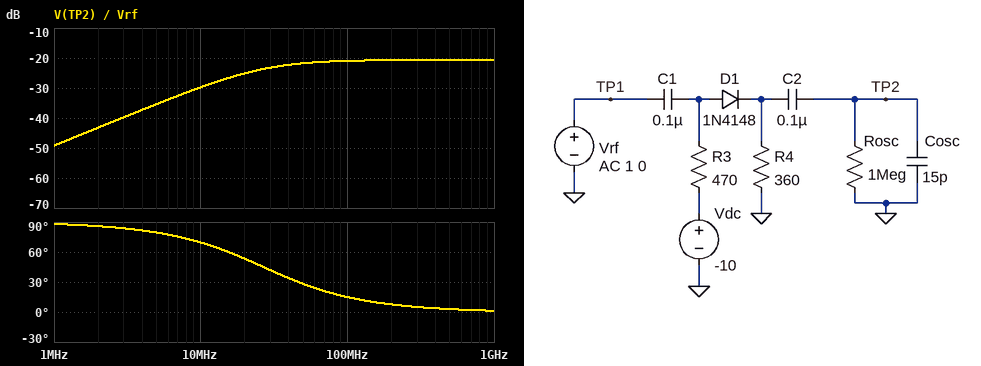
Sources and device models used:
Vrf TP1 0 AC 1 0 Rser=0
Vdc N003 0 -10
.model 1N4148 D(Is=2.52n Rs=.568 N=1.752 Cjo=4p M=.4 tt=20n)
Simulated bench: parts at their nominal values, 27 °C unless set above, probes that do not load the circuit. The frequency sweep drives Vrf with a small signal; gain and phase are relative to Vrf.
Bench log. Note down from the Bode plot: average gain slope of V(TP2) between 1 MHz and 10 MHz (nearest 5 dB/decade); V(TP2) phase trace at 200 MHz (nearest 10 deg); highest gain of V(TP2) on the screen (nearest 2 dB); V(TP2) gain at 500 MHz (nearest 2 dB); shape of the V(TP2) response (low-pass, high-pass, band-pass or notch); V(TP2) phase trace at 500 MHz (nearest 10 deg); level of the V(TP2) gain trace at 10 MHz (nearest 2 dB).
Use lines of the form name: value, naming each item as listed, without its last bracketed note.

average gain slope of V(TP2) between 1 MHz and 10 MHz: 20 dB/decade
V(TP2) phase trace at 200 MHz: 10 deg
highest gain of V(TP2) on the screen: -20 dB
V(TP2) gain at 500 MHz: -20 dB
shape of the V(TP2) response: high-pass
V(TP2) phase trace at 500 MHz: 0 deg
level of the V(TP2) gain trace at 10 MHz: -30 dB
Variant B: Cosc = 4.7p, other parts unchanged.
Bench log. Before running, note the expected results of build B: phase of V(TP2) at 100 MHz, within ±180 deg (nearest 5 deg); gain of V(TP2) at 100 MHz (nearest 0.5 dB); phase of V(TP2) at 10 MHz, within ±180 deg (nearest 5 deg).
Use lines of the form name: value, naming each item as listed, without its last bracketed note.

phase of V(TP2) at 100 MHz, within ±180 deg: 35 deg
gain of V(TP2) at 100 MHz: -14.0 dB
phase of V(TP2) at 10 MHz, within ±180 deg: 80 deg
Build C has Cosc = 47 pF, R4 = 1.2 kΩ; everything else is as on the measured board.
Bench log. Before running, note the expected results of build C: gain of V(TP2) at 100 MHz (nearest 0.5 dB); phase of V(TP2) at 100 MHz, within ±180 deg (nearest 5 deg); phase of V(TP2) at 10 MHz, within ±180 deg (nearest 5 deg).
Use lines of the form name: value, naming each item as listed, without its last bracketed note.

gain of V(TP2) at 100 MHz: -30.0 dB
phase of V(TP2) at 100 MHz, within ±180 deg: 0 deg
phase of V(TP2) at 10 MHz, within ±180 deg: 15 deg
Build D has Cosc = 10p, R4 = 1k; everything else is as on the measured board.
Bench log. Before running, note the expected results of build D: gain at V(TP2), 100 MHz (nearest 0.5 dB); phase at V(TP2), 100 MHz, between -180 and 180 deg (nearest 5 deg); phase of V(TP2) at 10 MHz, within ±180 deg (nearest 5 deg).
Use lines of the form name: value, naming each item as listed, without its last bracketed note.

gain at V(TP2), 100 MHz: -17.5 dB
phase at V(TP2), 100 MHz, between -180 and 180 deg: 10 deg
phase of V(TP2) at 10 MHz, within ±180 deg: 55 deg
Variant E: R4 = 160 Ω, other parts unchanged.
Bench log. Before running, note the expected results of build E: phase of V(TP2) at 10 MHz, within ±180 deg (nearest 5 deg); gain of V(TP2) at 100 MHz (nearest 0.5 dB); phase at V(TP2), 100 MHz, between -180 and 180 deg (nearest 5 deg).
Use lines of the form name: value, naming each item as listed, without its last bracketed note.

phase of V(TP2) at 10 MHz, within ±180 deg: 80 deg
gain of V(TP2) at 100 MHz: -22.0 dB
phase at V(TP2), 100 MHz, between -180 and 180 deg: 30 deg
